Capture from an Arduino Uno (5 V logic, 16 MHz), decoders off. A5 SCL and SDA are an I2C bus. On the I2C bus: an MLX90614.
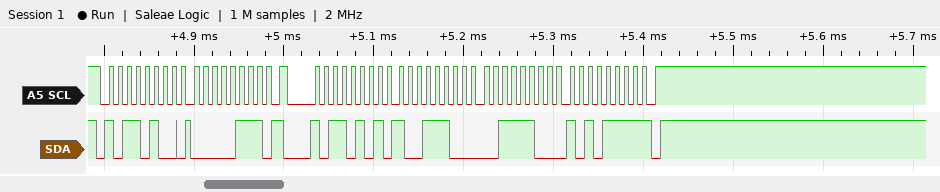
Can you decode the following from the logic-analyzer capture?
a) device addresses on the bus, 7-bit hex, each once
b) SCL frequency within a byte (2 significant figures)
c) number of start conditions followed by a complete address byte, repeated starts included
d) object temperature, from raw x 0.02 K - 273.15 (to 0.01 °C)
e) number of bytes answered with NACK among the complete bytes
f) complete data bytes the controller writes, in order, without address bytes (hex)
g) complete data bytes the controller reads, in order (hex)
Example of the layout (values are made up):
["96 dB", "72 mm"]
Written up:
["0x5A", "100 kHz", "2", "37.17 °C", "1", "07", "9C 3C AF"]
